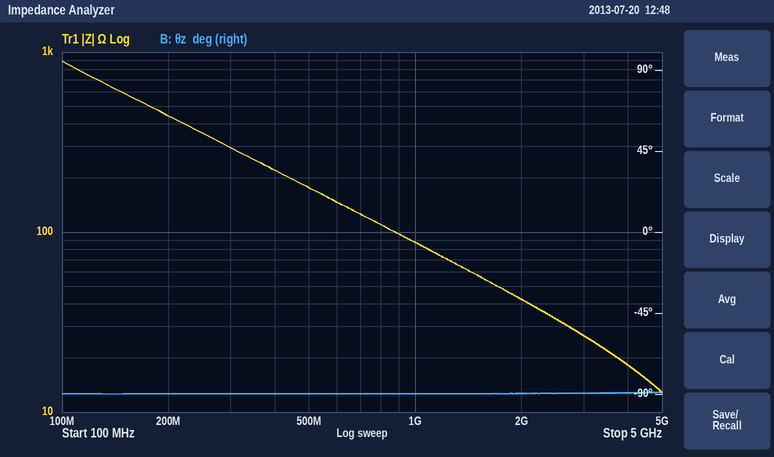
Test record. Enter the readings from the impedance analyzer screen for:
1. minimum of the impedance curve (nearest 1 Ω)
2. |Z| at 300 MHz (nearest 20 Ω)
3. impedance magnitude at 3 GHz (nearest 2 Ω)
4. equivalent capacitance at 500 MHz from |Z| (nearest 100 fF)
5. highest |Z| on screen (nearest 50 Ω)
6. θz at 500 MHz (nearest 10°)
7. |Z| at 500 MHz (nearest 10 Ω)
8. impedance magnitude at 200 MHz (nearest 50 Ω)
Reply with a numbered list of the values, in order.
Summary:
1. 13 Ω
2. 300 Ω
3. 26 Ω
4. 1.8 pF
5. 900 Ω
6. -90°
7. 180 Ω
8. 450 Ω
